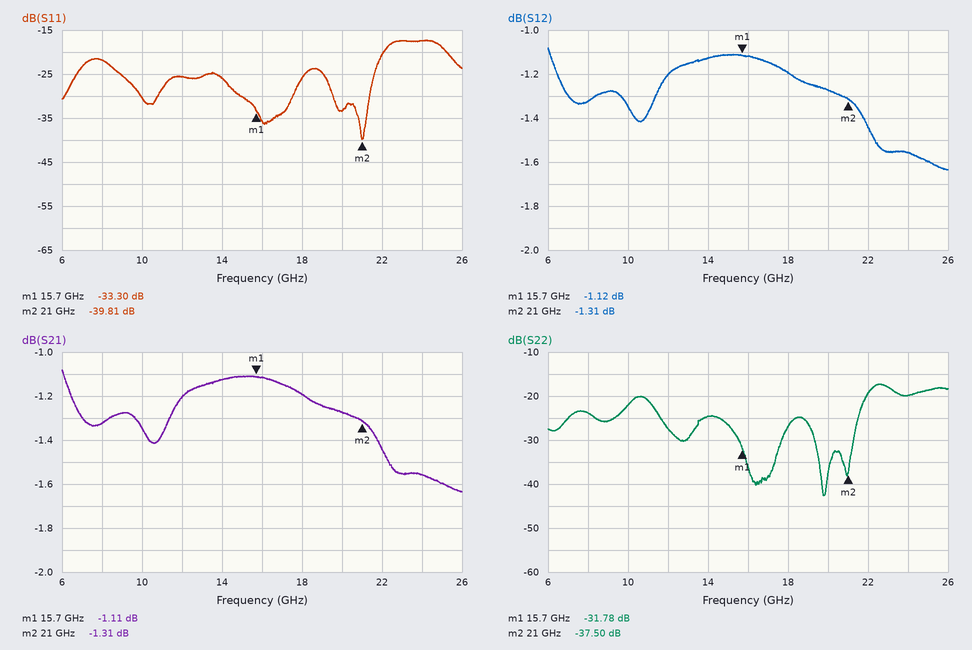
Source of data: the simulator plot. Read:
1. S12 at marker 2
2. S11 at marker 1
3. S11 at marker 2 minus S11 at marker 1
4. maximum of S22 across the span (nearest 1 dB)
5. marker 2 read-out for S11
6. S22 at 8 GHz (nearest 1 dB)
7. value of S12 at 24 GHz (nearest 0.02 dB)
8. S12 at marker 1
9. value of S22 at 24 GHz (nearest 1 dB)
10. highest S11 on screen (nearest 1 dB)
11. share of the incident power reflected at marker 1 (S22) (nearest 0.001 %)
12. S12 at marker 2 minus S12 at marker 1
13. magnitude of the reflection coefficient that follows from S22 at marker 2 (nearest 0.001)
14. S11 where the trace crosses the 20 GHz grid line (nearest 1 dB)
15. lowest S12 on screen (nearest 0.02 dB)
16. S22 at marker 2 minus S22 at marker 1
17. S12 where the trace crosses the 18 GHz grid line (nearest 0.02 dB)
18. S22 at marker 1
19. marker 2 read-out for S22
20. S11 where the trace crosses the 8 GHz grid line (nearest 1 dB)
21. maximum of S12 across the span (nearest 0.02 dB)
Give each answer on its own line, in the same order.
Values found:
-1.31 dB
-33.30 dB
-6.51 dB
-17 dB
-39.81 dB
-24 dB
-1.56 dB
-1.12 dB
-20 dB
-17 dB
0.066 %
-0.19 dB
0.013
-33 dB
-1.64 dB
-5.72 dB
-1.20 dB
-31.78 dB
-37.50 dB
-22 dB
-1.08 dB
